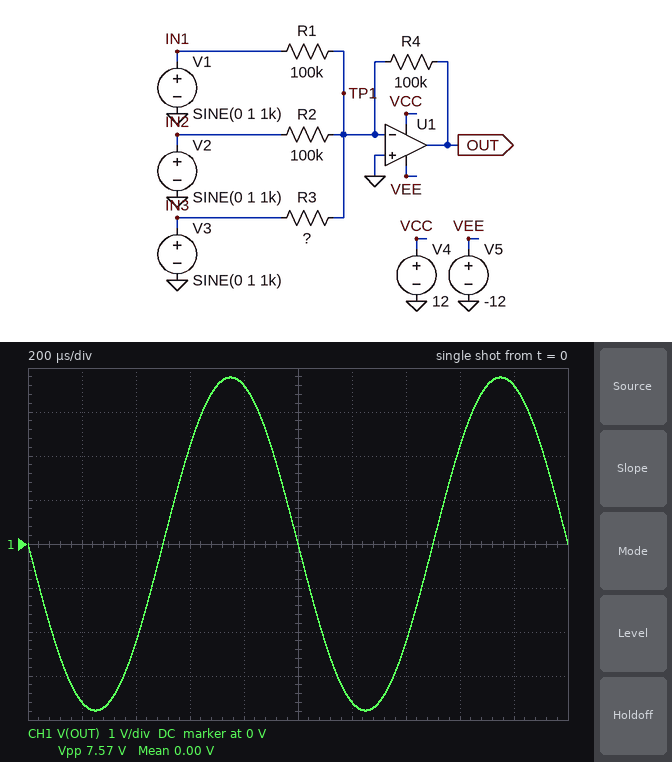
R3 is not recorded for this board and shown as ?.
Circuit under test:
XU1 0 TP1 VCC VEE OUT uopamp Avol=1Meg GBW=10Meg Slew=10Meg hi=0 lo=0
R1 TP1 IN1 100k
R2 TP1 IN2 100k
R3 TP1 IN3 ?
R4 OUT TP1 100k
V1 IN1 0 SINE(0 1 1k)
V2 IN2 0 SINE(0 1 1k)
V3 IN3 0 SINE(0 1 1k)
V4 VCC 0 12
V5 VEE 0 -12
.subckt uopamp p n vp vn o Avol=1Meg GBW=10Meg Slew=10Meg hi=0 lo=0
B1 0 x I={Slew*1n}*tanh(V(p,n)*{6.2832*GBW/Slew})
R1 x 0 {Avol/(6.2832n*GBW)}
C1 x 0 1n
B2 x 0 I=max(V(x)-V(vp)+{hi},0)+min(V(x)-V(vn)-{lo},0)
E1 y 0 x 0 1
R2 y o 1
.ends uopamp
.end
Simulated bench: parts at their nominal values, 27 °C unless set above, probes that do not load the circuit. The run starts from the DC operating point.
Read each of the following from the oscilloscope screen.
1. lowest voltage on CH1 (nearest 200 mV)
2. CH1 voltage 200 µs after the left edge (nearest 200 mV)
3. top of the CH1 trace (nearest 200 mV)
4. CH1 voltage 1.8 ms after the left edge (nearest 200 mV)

-3.8 V
-3.6 V
3.8 V
3.6 V
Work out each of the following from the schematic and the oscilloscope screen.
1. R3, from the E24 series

56 kΩ
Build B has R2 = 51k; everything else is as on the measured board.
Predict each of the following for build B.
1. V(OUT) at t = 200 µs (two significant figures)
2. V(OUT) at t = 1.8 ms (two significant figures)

-4.5 V
4.5 V
